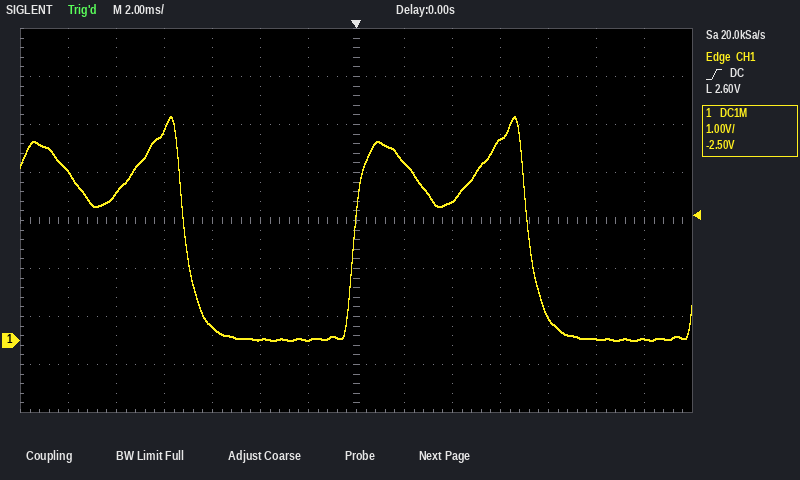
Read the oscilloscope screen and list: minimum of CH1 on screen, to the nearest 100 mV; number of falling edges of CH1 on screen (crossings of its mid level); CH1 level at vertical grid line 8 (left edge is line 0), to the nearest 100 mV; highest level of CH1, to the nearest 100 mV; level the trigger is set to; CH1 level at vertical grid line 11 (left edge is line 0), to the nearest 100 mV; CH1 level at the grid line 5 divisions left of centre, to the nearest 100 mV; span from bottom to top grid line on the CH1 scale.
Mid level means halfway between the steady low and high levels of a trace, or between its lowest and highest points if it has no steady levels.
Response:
0.0 V
2
3.7 V
4.7 V
2.60 V
500 mV
3.1 V
8 V
